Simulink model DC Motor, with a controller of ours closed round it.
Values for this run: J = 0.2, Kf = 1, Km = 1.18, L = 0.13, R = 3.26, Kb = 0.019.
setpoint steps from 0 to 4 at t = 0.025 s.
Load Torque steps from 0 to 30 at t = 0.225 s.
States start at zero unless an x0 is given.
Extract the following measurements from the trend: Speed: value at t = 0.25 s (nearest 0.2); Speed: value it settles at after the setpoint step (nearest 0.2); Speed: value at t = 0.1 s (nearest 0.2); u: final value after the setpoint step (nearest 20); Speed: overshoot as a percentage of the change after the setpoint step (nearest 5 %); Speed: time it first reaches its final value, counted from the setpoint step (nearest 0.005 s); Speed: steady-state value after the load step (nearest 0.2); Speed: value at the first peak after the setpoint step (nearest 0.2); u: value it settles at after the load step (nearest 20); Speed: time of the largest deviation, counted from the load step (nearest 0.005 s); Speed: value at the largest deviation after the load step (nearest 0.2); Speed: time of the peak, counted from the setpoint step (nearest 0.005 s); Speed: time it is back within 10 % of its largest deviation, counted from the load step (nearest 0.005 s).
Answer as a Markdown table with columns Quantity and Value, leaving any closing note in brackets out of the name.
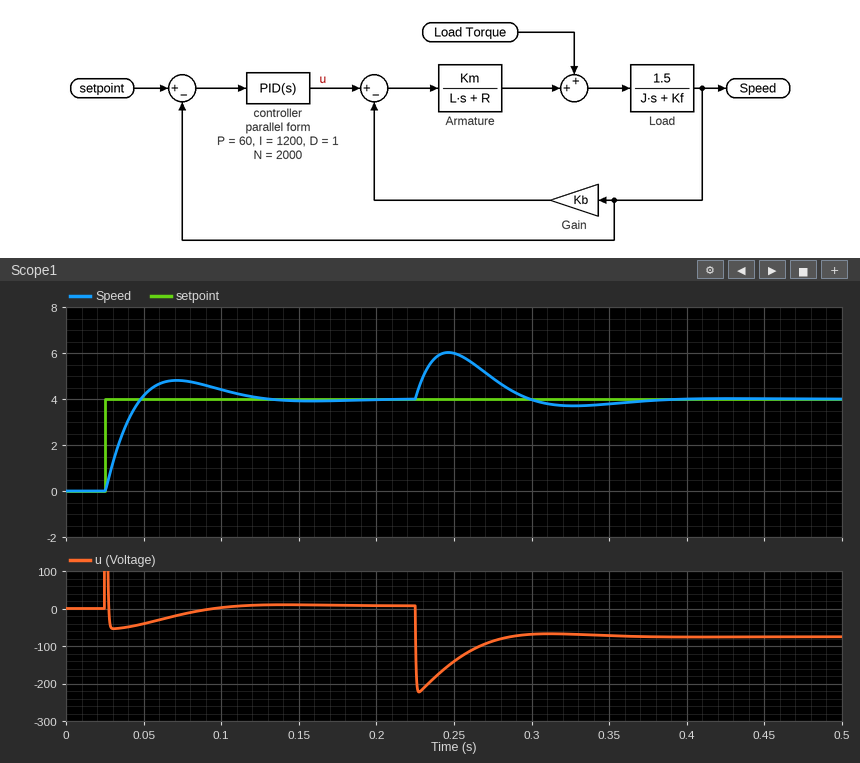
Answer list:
| Quantity | Value |
|---|---|
| Speed: value at t = 0.25 s | 6.0 |
| Speed: value it settles at after the setpoint step | 4.0 |
| Speed: value at t = 0.1 s | 4.4 |
| u: final value after the setpoint step | 0 |
| Speed: overshoot as a percentage of the change after the setpoint step | 20 % |
| Speed: time it first reaches its final value, counted from the setpoint step | 0.025 s |
| Speed: steady-state value after the load step | 4.0 |
| Speed: value at the first peak after the setpoint step | 4.8 |
| u: value it settles at after the load step | -80 |
| Speed: time of the largest deviation, counted from the load step | 0.020 s |
| Speed: value at the largest deviation after the load step | 6.0 |
| Speed: time of the peak, counted from the setpoint step | 0.045 s |
| Speed: time it is back within 10 % of its largest deviation, counted from the load step | 0.125 s |
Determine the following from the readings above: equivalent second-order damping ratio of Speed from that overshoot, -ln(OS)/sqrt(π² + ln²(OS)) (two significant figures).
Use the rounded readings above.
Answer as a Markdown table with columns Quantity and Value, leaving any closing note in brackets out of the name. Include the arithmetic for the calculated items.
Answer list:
| Quantity | Value |
|---|---|
| equivalent second-order damping ratio of Speed from that overshoot, -ln(OS)/sqrt(π² + ln²(OS)) | ln(0.2) = -1.609; 1.609 / sqrt(9.870 + 2.590) = 0.46 |
